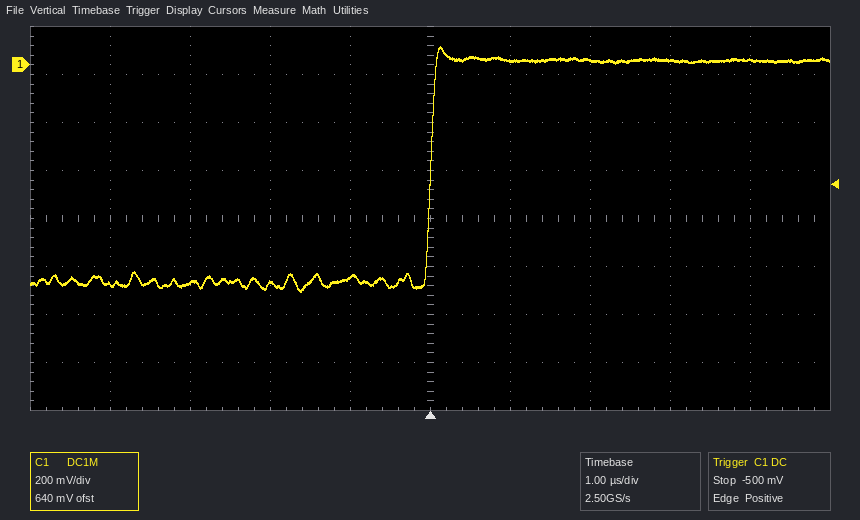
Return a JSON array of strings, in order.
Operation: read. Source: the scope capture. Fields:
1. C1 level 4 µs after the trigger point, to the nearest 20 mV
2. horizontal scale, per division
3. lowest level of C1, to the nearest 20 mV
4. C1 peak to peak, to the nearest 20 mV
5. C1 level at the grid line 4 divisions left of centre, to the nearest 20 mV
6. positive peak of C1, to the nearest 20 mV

["20 mV", "1 µs", "-940 mV", "1.02 V", "-920 mV", "80 mV"]
